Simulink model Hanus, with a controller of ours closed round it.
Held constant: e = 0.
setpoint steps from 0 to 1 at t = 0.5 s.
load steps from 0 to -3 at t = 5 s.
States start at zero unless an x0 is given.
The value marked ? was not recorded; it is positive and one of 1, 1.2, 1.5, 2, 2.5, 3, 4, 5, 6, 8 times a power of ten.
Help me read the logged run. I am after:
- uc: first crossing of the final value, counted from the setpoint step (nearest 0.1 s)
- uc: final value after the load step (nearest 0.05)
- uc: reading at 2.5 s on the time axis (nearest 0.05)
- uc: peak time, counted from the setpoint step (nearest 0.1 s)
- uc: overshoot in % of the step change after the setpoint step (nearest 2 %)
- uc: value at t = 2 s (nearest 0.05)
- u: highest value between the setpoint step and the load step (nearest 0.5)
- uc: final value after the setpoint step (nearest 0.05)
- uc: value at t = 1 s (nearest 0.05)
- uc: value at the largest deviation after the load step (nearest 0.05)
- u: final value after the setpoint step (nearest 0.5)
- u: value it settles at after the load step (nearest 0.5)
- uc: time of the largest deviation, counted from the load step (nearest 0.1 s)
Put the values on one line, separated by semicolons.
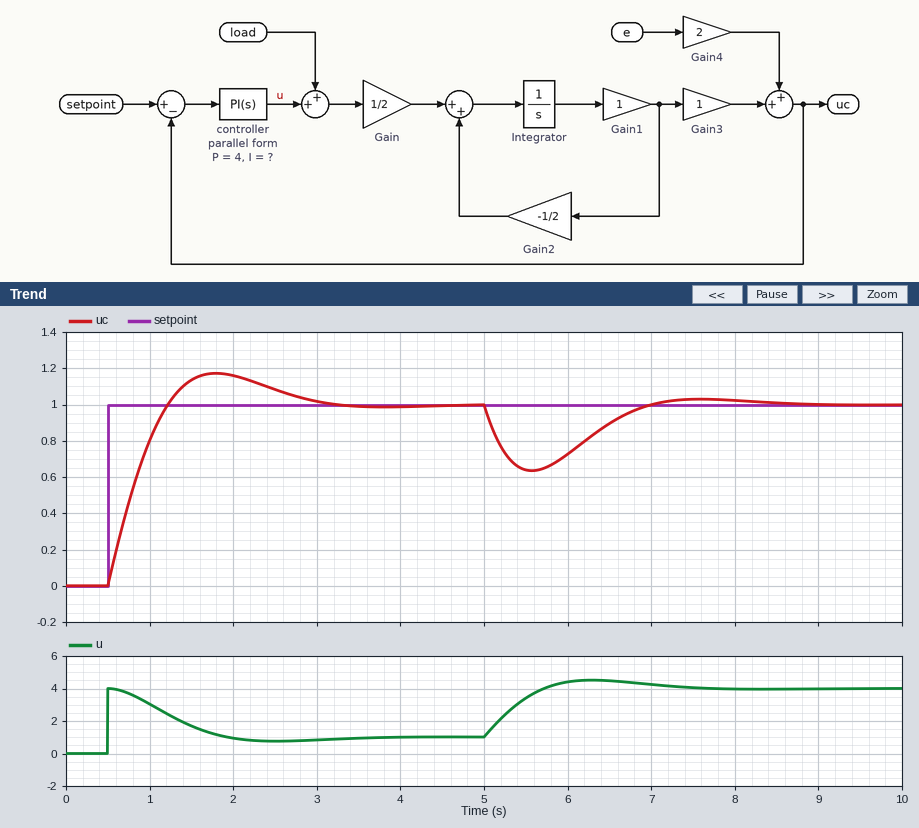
0.7 s; 1.00; 1.10; 1.3 s; 18 %; 1.15; 4.0; 1.00; 0.80; 0.65; 1.0; 4.0; 0.6 s
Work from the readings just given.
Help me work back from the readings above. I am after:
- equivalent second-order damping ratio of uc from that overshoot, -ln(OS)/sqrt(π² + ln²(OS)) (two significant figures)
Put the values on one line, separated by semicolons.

0.48
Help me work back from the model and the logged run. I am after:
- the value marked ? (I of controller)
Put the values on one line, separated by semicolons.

8
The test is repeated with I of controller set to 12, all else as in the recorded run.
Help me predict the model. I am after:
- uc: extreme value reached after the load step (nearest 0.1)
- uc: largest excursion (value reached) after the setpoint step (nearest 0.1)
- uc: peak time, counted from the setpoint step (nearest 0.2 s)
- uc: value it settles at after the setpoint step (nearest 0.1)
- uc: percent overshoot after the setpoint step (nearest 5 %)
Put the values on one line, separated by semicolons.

0.7; 1.2; 1.0 s; 1.0; 25 %
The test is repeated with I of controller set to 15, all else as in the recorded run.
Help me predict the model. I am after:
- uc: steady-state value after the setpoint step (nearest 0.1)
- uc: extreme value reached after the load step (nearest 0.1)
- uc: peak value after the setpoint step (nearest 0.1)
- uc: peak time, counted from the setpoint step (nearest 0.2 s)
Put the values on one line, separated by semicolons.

1.0; 0.7; 1.3; 1.0 s
